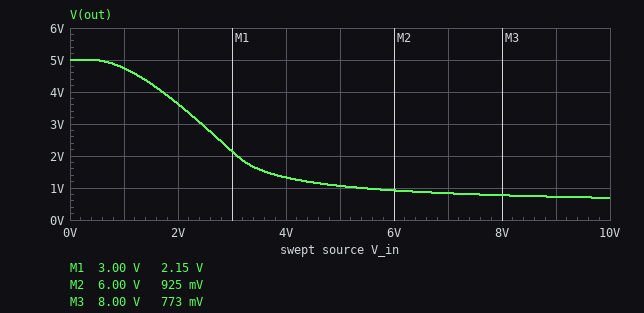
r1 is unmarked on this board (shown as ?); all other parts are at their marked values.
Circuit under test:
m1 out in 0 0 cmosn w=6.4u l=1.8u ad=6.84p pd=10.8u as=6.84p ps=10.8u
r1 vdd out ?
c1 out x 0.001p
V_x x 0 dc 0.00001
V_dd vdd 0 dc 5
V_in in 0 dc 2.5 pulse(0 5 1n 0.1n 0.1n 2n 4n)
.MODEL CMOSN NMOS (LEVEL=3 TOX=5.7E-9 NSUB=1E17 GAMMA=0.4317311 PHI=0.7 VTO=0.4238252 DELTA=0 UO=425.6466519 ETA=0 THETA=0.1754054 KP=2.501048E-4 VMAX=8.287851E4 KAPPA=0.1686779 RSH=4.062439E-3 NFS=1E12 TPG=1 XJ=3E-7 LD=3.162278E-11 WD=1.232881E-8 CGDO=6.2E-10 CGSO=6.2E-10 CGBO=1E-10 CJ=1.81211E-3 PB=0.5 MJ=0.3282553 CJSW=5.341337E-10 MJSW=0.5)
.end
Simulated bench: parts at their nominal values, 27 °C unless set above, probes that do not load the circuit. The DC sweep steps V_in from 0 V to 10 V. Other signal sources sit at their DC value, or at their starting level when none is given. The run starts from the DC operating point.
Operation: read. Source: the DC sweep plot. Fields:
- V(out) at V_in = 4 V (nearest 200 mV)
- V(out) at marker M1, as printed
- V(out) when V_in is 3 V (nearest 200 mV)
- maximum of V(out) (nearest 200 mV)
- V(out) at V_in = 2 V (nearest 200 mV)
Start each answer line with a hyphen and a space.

- 1.4 V
- 2.15 V
- 2.2 V
- 5.0 V
- 3.6 V
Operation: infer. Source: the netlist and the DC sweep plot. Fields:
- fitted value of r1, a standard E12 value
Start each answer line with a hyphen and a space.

- 2.2 kΩ
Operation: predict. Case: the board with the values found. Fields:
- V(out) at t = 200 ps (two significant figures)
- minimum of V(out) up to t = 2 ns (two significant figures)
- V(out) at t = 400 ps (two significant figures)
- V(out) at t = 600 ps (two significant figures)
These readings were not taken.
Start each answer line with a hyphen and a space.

- 5.0 V
- 1.1 V
- 5.0 V
- 5.0 V
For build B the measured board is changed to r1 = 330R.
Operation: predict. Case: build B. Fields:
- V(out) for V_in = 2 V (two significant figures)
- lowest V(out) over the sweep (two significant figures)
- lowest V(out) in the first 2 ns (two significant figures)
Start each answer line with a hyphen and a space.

- 4.8 V
- 3.0 V
- 4.0 V
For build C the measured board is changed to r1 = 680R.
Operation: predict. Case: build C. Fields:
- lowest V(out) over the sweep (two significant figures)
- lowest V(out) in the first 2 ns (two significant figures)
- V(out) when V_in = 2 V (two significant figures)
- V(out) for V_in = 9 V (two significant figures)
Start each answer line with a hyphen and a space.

- 1.9 V
- 3.0 V
- 4.6 V
- 2.0 V
